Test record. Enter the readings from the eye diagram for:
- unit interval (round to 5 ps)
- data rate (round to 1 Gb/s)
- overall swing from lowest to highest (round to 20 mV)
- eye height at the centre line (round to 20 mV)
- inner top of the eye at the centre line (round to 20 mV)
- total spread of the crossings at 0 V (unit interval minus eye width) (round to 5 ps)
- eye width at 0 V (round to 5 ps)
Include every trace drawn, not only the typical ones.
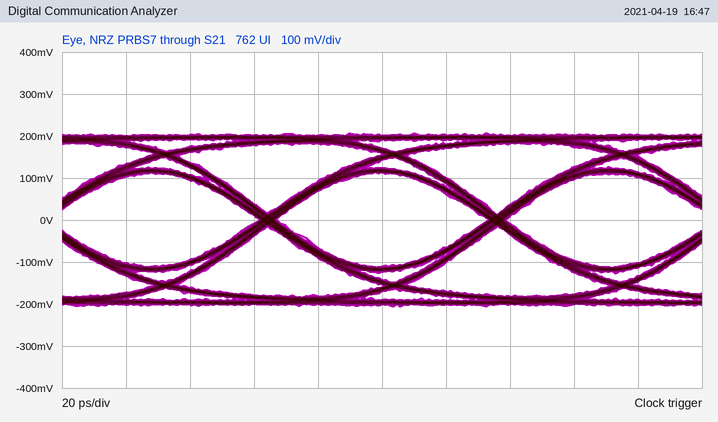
70 ps
14 Gb/s
420 mV
220 mV
120 mV
5 ps
65 ps
